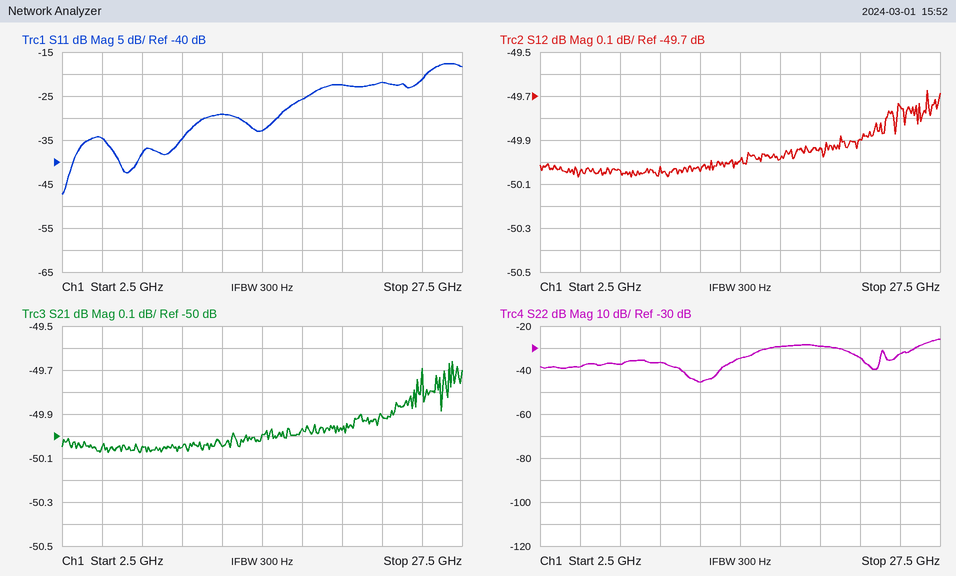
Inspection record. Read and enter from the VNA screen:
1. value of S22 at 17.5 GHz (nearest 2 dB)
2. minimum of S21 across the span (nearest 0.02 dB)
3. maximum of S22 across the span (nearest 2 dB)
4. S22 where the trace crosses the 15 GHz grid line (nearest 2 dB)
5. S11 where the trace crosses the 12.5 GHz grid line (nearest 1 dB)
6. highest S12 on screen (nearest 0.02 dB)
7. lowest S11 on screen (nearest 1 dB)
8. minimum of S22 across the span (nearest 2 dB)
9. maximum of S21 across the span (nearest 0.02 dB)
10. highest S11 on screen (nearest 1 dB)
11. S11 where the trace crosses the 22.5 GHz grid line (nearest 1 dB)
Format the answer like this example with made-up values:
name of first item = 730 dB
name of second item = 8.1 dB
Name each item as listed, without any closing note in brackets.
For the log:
value of S22 at 17.5 GHz = -30 dB
minimum of S21 across the span = -50.08 dB
maximum of S22 across the span = -26 dB
S22 where the trace crosses the 15 GHz grid line = -34 dB
S11 where the trace crosses the 12.5 GHz grid line = -29 dB
highest S12 on screen = -49.68 dB
lowest S11 on screen = -47 dB
minimum of S22 across the span = -46 dB
maximum of S21 across the span = -49.66 dB
highest S11 on screen = -18 dB
S11 where the trace crosses the 22.5 GHz grid line = -22 dB
